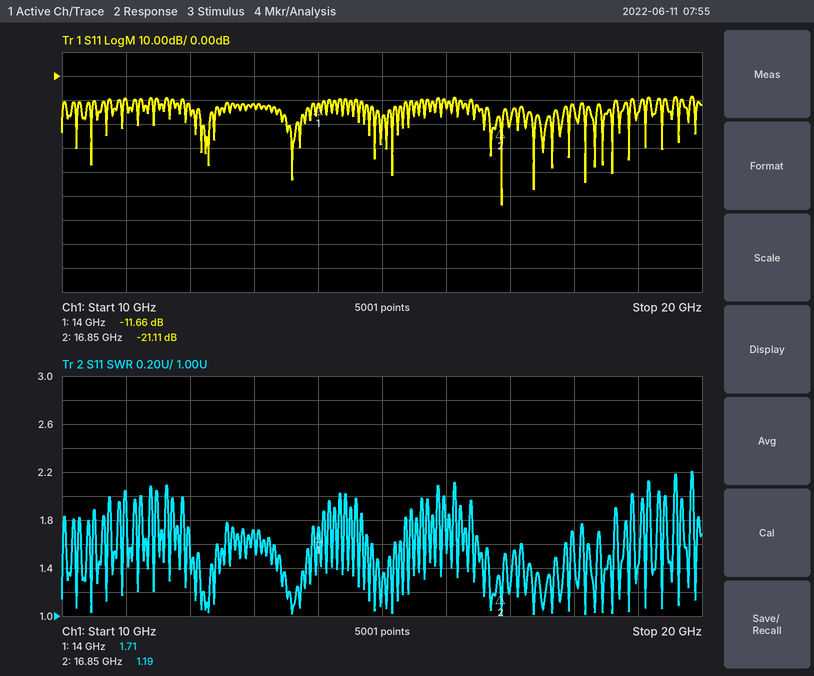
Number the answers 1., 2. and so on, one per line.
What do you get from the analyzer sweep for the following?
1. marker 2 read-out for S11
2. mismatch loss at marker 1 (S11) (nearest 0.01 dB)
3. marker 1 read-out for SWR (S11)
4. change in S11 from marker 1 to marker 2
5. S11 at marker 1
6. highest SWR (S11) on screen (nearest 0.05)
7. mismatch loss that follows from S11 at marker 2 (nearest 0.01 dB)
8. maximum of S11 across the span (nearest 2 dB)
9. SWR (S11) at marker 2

1. -21.11 dB
2. 0.31 dB
3. 1.71
4. -9.45 dB
5. -11.66 dB
6. 2.20
7. 0.03 dB
8. -8 dB
9. 1.19
